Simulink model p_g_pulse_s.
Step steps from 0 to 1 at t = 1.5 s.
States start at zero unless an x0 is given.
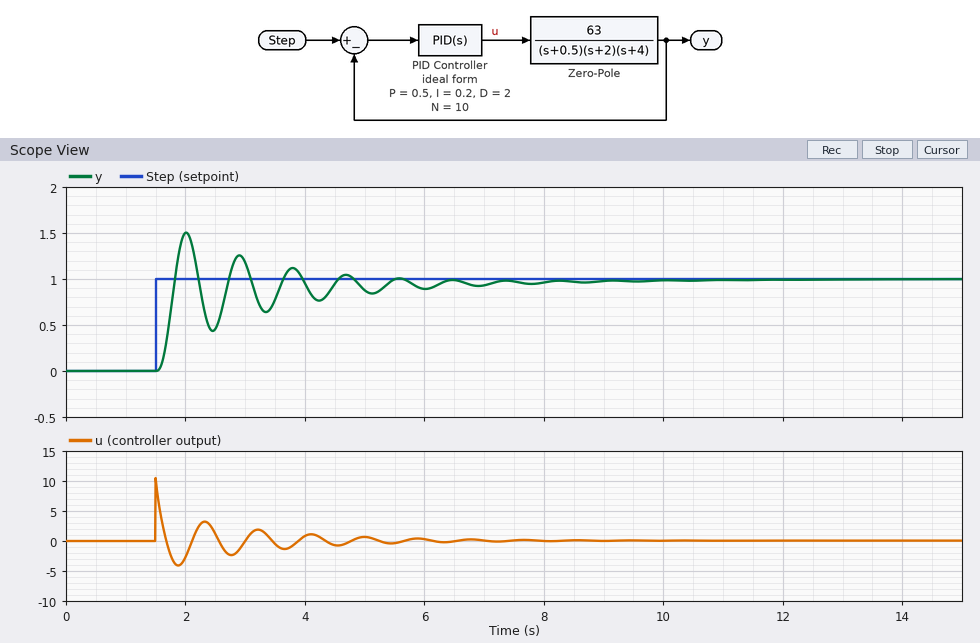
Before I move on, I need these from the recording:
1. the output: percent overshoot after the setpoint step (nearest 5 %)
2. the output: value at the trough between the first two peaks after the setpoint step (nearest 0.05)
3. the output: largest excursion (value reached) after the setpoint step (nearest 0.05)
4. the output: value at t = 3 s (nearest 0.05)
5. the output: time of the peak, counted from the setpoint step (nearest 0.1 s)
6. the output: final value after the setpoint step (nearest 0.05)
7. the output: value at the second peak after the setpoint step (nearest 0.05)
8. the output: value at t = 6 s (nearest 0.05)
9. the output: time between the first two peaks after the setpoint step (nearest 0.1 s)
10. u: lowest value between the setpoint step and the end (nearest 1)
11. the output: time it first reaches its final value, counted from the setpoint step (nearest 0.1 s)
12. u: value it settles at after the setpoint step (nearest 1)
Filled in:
50 %
0.45
1.50
1.20
0.5 s
1.00
1.25
0.90
0.9 s
-4
0.3 s
0
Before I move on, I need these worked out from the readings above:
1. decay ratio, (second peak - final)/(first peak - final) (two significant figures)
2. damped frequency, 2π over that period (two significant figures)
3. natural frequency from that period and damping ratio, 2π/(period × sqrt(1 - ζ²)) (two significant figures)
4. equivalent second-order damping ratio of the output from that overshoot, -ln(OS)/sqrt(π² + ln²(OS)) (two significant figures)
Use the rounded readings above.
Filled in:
0.50
7.0 rad/s
7.2 rad/s
0.22
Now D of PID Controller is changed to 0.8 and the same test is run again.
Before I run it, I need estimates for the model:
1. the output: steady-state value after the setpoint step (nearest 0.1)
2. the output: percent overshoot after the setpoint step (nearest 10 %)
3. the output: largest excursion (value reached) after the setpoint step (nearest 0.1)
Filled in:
1.0
20 %
1.2
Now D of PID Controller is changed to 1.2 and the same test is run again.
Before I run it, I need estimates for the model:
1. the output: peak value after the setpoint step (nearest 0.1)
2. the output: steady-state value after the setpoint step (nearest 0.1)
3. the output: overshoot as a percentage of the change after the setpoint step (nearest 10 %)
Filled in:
1.3
1.0
30 %
